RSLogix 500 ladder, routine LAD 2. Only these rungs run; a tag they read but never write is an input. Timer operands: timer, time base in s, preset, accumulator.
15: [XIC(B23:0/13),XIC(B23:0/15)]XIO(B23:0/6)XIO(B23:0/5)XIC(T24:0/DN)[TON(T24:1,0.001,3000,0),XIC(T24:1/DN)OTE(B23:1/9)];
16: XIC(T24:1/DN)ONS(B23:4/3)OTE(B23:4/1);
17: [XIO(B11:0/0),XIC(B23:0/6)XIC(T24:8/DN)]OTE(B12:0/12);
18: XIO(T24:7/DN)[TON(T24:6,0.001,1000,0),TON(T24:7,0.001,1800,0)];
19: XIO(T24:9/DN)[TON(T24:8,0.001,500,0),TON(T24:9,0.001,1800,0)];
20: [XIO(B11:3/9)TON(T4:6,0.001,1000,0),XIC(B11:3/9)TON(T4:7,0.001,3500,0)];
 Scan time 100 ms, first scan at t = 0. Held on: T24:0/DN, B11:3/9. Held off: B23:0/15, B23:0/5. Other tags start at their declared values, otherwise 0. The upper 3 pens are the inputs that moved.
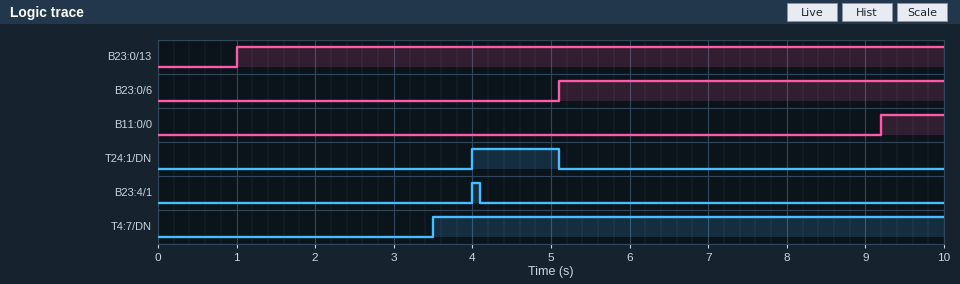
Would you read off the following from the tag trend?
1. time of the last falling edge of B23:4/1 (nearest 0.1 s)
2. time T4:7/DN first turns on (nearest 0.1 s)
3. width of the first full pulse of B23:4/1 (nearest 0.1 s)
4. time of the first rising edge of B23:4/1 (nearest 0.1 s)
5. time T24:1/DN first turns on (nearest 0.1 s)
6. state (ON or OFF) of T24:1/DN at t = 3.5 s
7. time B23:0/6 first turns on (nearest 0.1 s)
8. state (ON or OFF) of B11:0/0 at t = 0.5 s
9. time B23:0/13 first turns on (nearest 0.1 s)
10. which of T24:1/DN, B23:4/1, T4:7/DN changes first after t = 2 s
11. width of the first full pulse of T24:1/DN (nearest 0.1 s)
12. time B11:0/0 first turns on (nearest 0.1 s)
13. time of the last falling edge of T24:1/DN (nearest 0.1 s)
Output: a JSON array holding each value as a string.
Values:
["4.1 s", "3.5 s", "0.1 s", "4.0 s", "4.0 s", "OFF", "5.1 s", "OFF", "1.0 s", "T4:7/DN", "1.1 s", "9.2 s", "5.1 s"]
